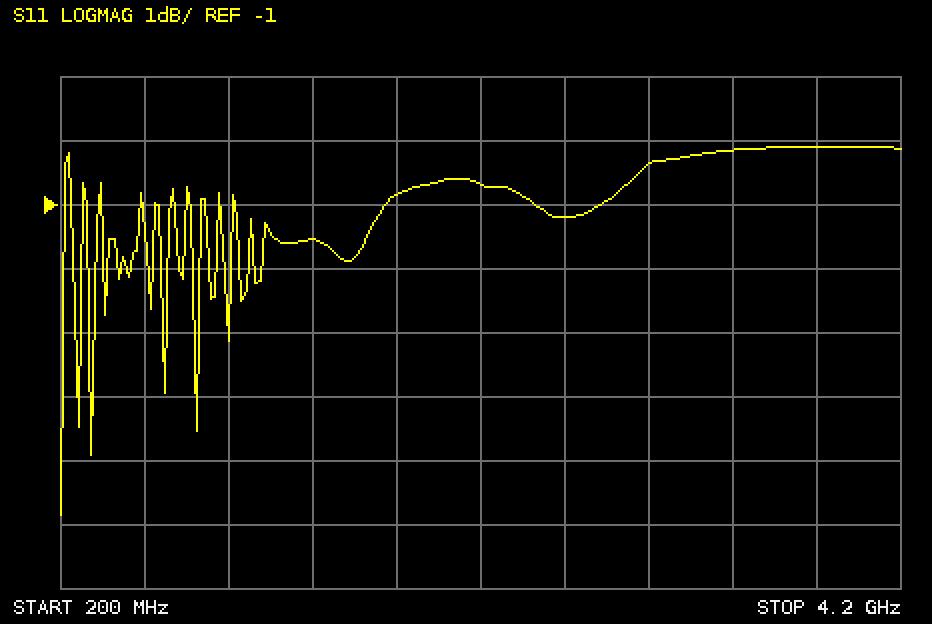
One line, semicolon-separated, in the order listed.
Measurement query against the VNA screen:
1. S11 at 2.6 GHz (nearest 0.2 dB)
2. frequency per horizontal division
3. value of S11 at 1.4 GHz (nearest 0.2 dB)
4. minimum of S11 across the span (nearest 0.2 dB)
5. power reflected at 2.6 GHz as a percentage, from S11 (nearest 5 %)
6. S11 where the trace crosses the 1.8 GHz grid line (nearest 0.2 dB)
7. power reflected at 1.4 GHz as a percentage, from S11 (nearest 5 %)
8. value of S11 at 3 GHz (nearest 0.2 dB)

-1.2 dB; 400 MHz; -1.6 dB; -5.8 dB; 75 %; -0.8 dB; 70 %; -0.4 dB
